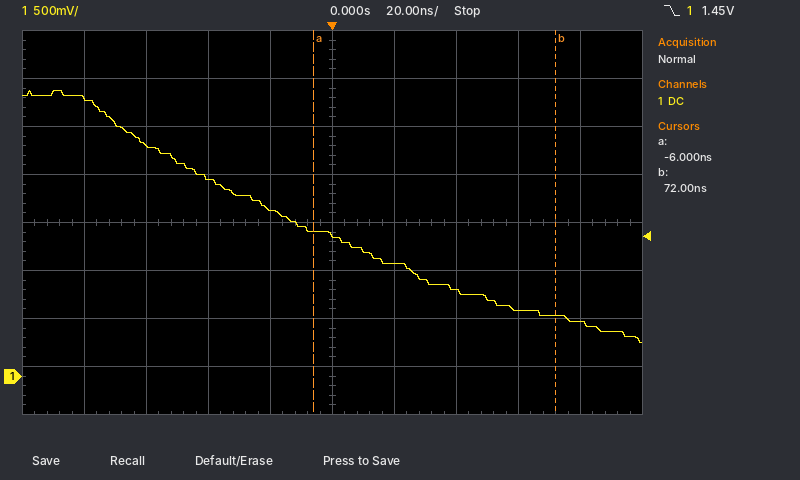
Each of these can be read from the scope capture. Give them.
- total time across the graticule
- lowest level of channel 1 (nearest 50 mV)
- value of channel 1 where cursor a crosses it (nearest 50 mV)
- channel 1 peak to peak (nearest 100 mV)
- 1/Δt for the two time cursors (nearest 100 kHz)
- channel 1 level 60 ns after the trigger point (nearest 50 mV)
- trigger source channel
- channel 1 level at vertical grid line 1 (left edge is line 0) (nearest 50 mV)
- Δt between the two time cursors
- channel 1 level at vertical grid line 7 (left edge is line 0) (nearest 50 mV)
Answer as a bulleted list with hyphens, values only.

- 200 ns
- 350 mV
- 1.50 V
- 2.60 V
- 12.8 MHz
- 700 mV
- channel 1
- 2.90 V
- 78 ns
- 900 mV
